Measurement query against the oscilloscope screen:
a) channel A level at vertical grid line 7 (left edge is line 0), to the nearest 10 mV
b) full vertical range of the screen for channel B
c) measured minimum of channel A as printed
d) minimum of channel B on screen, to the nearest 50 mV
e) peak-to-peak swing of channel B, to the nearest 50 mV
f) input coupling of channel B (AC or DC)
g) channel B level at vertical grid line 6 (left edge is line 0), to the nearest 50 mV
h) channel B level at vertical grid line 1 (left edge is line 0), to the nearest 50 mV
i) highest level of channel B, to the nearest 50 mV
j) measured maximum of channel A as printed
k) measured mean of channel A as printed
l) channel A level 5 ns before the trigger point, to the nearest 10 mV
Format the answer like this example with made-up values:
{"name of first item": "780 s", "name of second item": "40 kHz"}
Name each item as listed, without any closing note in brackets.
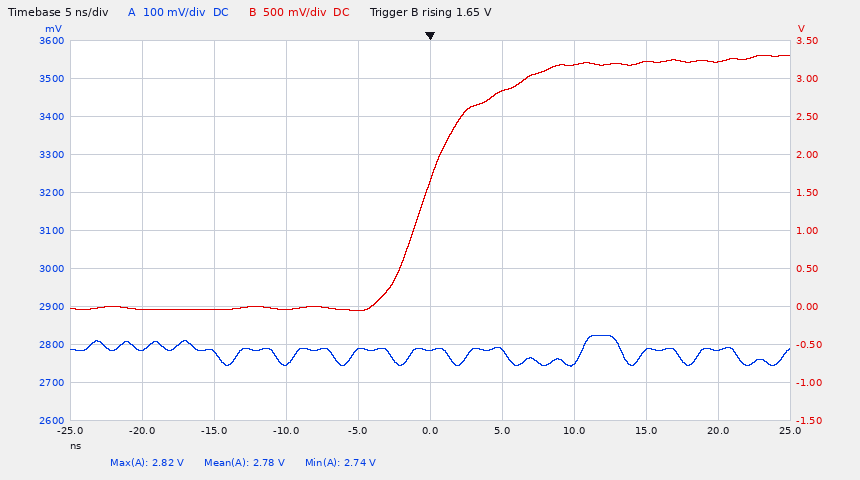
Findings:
{"channel A level at vertical grid line 7 (left edge is line 0), to the nearest 10 mV": "2.75 V", "full vertical range of the screen for channel B": "5 V", "measured minimum of channel A as printed": "2.74 V", "minimum of channel B on screen, to the nearest 50 mV": "-50 mV", "peak-to-peak swing of channel B, to the nearest 50 mV": "3.35 V", "input coupling of channel B": "DC", "channel B level at vertical grid line 6 (left edge is line 0), to the nearest 50 mV": "2.85 V", "channel B level at vertical grid line 1 (left edge is line 0), to the nearest 50 mV": "-50 mV", "highest level of channel B, to the nearest 50 mV": "3.30 V", "measured maximum of channel A as printed": "2.82 V", "measured mean of channel A as printed": "2.78 V", "channel A level 5 ns before the trigger point, to the nearest 10 mV": "2.79 V"}
